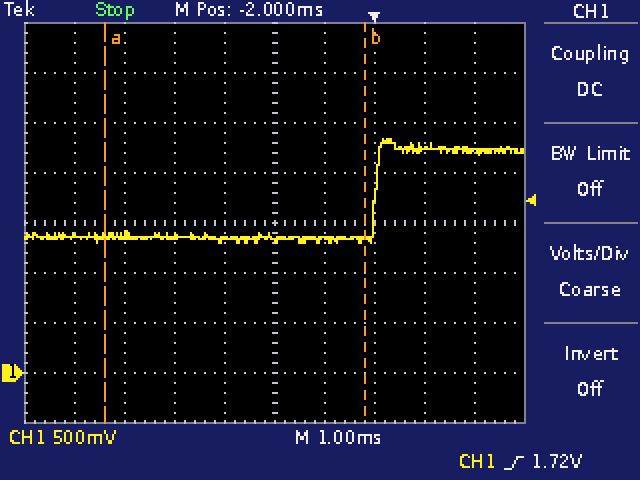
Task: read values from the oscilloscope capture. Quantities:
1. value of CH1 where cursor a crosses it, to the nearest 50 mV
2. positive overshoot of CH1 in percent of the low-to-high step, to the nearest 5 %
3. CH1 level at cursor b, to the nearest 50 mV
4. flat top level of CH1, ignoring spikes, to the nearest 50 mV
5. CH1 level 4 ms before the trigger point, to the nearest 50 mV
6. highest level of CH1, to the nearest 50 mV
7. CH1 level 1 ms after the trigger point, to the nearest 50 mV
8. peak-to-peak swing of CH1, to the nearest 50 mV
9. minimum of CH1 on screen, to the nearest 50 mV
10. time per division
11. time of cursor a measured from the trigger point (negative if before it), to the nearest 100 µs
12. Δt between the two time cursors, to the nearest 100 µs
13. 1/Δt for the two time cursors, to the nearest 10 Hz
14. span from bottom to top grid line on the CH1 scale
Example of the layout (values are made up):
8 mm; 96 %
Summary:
1.35 V; 10 %; 1.35 V; 2.25 V; 1.35 V; 2.35 V; 2.25 V; 1.05 V; 1.30 V; 1 ms; -5.4 ms; 5.2 ms; 190 Hz; 4 V
